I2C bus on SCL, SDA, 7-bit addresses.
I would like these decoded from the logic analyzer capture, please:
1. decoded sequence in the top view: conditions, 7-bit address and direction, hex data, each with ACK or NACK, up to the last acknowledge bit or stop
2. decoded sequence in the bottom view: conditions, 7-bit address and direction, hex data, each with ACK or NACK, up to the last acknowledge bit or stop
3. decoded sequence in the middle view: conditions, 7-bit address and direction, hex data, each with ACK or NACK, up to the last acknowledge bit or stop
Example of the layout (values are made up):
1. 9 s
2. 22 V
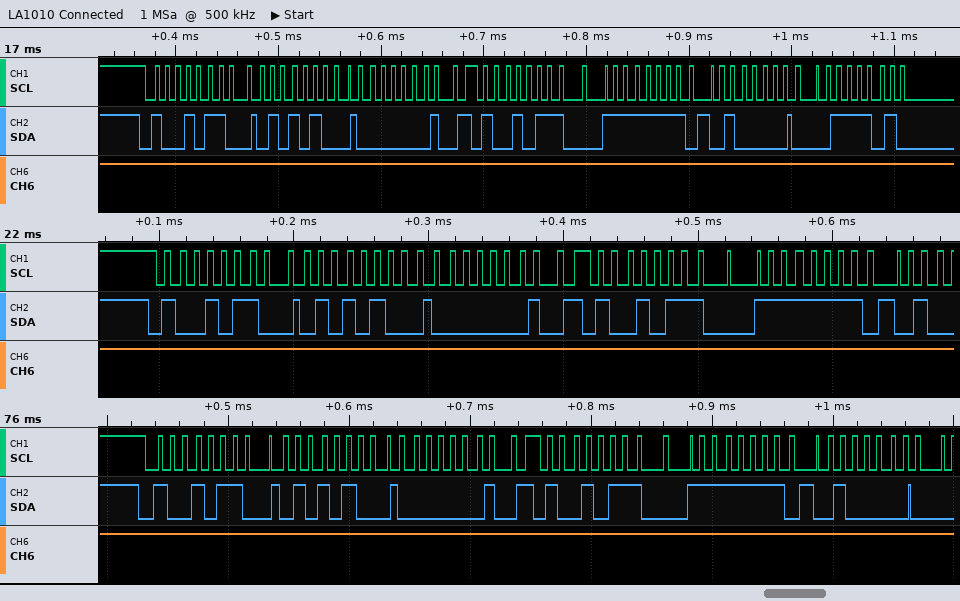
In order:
1. start, address 4B write ACK, 54 ACK, 01 ACK, repeated start, address 4B read ACK, FF ACK, 20 ACK, 3D ACK
2. start, address 4B write ACK, 54 ACK, 01 ACK, repeated start, address 4B read ACK, FF ACK, 20 ACK
3. start, address 4B write ACK, 54 ACK, 01 ACK, repeated start, address 4B read ACK, FF ACK
